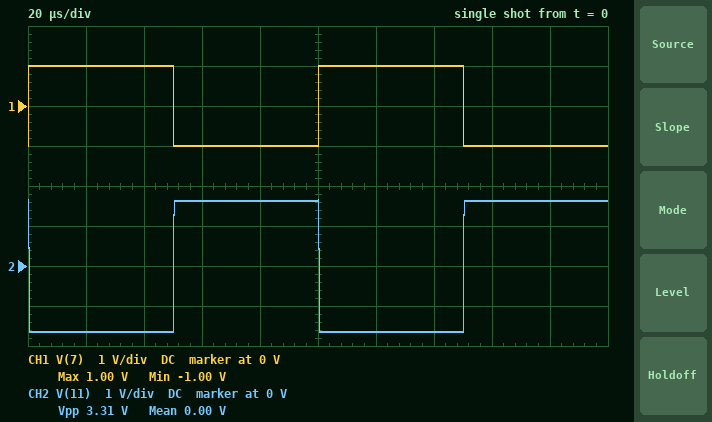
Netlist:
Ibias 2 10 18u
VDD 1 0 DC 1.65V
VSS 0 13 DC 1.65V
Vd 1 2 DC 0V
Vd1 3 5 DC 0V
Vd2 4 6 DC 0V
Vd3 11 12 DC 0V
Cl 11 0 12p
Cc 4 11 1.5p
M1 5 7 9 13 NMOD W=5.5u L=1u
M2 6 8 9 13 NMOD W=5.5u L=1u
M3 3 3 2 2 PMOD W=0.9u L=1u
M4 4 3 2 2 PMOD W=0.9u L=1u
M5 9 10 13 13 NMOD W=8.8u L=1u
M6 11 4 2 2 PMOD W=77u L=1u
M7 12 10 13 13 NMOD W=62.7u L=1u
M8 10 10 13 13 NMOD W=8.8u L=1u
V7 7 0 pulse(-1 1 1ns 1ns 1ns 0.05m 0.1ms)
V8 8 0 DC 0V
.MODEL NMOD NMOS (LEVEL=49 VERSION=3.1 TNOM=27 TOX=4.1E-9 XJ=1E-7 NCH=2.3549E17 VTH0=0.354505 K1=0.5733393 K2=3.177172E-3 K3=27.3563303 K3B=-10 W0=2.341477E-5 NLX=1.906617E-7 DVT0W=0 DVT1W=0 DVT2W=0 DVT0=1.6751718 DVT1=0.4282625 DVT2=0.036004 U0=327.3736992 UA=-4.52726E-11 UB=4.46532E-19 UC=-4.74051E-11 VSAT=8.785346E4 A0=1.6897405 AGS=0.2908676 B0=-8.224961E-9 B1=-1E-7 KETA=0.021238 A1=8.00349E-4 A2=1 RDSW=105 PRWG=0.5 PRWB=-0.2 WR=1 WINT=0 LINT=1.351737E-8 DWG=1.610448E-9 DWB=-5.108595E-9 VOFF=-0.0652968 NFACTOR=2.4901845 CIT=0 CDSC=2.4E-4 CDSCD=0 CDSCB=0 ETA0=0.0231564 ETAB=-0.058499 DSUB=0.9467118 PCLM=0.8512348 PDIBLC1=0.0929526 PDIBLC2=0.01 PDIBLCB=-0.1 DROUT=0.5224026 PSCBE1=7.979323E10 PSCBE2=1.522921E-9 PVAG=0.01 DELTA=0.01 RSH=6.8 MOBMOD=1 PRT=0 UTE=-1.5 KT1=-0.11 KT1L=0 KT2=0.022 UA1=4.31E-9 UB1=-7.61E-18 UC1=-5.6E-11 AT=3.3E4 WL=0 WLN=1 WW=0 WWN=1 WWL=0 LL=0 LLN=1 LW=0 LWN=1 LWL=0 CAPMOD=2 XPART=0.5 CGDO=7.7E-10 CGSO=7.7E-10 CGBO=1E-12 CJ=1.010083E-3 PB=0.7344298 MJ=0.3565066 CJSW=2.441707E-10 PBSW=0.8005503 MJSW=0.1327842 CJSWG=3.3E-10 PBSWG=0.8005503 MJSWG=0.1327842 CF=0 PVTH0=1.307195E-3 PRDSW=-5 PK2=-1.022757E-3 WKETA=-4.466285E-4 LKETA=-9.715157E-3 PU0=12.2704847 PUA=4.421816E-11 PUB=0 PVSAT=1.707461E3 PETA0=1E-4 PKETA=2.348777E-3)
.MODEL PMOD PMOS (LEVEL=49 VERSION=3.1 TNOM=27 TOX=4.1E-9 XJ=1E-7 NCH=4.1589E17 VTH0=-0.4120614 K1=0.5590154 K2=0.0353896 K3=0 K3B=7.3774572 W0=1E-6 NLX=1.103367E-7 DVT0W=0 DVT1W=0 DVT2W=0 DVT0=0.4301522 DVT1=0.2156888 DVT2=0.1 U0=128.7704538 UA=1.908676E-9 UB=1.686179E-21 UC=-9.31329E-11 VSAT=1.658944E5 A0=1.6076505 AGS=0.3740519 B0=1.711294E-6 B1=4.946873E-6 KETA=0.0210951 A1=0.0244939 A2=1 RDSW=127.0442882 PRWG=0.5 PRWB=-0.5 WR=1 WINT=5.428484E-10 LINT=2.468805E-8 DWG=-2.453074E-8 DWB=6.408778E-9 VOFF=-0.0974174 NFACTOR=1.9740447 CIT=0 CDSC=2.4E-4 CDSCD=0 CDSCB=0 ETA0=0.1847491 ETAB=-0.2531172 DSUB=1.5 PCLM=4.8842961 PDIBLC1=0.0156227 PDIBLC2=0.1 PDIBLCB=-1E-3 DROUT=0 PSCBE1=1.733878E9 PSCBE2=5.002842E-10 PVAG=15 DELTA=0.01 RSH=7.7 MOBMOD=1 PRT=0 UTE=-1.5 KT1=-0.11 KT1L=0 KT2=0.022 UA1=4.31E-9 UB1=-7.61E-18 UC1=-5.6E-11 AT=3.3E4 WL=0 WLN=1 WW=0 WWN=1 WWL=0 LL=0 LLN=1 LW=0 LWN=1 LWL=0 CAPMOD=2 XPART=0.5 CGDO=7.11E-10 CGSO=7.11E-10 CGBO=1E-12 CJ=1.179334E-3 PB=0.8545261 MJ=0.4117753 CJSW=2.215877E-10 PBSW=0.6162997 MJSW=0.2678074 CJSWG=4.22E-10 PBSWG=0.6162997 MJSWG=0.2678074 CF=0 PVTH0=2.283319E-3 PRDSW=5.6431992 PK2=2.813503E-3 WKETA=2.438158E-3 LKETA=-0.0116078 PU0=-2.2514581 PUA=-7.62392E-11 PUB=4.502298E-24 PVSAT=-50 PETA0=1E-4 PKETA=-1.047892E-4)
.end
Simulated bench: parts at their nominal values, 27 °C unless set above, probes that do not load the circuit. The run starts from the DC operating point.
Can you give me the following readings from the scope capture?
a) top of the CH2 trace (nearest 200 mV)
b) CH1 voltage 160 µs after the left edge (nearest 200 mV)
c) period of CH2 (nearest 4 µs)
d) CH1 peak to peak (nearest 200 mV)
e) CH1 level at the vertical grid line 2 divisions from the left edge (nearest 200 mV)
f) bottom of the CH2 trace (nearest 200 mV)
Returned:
1.6 V
-1.0 V
100 µs
2.0 V
1.0 V
-1.6 V
